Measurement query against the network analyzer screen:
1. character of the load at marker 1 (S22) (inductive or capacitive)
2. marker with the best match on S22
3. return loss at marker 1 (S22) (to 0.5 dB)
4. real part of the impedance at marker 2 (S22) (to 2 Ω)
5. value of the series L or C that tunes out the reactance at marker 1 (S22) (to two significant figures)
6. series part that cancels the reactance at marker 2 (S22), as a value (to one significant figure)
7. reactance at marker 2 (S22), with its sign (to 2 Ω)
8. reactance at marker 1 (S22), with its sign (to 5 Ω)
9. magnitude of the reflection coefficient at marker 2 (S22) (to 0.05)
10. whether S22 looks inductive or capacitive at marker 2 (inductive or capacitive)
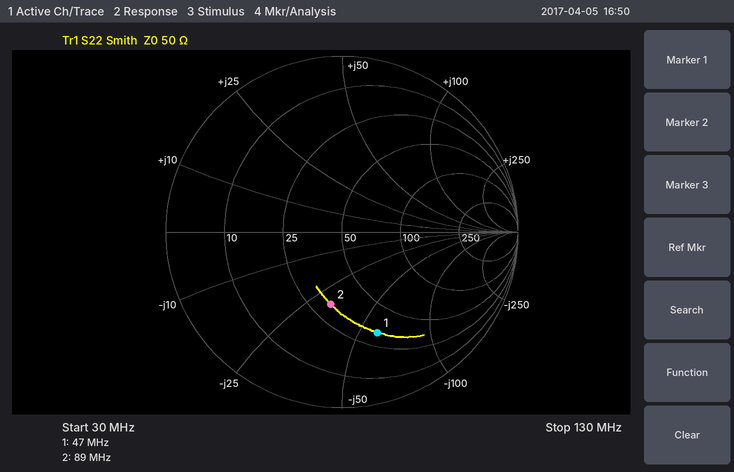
capacitive
marker 2
4.5 dB
32 Ω
200 nH
60 nH
-32 Ω
-60 Ω
0.40
capacitive
